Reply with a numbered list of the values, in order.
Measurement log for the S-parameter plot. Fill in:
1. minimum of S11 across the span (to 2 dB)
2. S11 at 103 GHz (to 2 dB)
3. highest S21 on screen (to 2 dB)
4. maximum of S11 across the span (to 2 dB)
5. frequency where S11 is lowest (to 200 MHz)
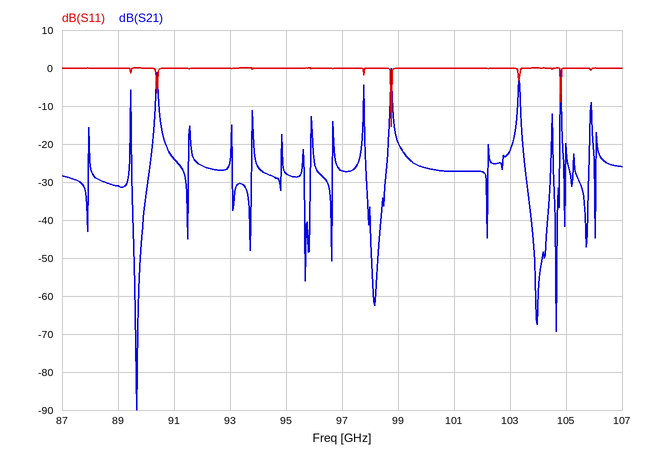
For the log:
1. -16 dB
2. 0 dB
3. 0 dB
4. 0 dB
5. 98.8 GHz
